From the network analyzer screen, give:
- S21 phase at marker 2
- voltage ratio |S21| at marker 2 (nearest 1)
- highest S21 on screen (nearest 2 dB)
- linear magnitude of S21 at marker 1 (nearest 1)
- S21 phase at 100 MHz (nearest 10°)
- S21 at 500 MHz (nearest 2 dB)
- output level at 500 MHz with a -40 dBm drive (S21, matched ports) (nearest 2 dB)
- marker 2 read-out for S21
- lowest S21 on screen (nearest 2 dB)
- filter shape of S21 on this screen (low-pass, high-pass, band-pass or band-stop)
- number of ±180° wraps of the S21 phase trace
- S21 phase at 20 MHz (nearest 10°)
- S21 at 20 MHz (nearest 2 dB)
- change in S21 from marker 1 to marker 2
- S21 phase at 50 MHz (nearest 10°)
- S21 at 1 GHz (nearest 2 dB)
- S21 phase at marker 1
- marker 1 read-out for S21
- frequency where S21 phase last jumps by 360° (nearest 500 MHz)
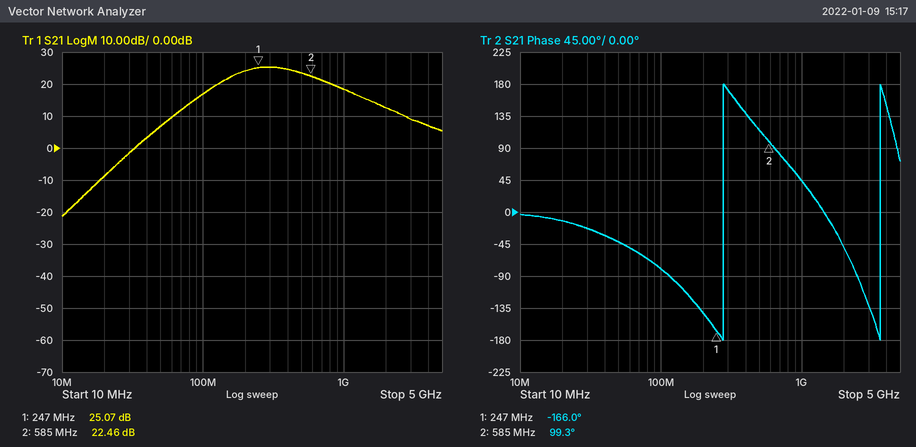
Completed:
99.3°
13
26 dB
18
-80°
24 dB
-16 dBm
22.46 dB
-22 dB
band-pass
2
-10°
-8 dB
-2.61 dB
-40°
18 dB
-166.0°
25.07 dB
3.5 GHz
